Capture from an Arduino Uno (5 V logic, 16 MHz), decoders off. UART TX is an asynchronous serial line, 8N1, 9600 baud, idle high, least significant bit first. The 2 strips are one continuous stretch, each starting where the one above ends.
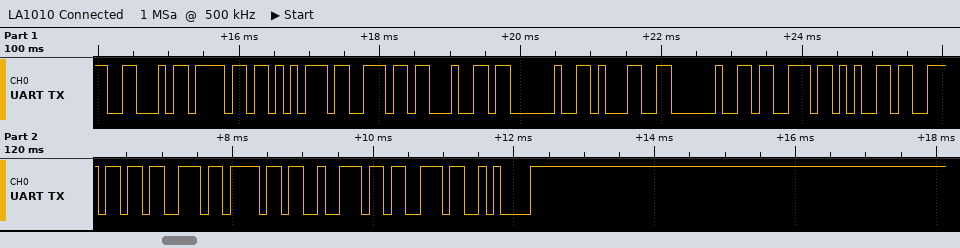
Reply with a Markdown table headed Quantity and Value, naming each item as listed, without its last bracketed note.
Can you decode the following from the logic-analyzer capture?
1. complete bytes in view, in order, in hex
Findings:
| Quantity | Value |
|---|---|
| complete bytes in view, in order, in hex | 0x46 0x6F 0x75 0x6E 0x64 0x20 0x31 0x20 0x73 0x65 0x6E 0x73 0x6F 0x72 0x73 0x0A |
